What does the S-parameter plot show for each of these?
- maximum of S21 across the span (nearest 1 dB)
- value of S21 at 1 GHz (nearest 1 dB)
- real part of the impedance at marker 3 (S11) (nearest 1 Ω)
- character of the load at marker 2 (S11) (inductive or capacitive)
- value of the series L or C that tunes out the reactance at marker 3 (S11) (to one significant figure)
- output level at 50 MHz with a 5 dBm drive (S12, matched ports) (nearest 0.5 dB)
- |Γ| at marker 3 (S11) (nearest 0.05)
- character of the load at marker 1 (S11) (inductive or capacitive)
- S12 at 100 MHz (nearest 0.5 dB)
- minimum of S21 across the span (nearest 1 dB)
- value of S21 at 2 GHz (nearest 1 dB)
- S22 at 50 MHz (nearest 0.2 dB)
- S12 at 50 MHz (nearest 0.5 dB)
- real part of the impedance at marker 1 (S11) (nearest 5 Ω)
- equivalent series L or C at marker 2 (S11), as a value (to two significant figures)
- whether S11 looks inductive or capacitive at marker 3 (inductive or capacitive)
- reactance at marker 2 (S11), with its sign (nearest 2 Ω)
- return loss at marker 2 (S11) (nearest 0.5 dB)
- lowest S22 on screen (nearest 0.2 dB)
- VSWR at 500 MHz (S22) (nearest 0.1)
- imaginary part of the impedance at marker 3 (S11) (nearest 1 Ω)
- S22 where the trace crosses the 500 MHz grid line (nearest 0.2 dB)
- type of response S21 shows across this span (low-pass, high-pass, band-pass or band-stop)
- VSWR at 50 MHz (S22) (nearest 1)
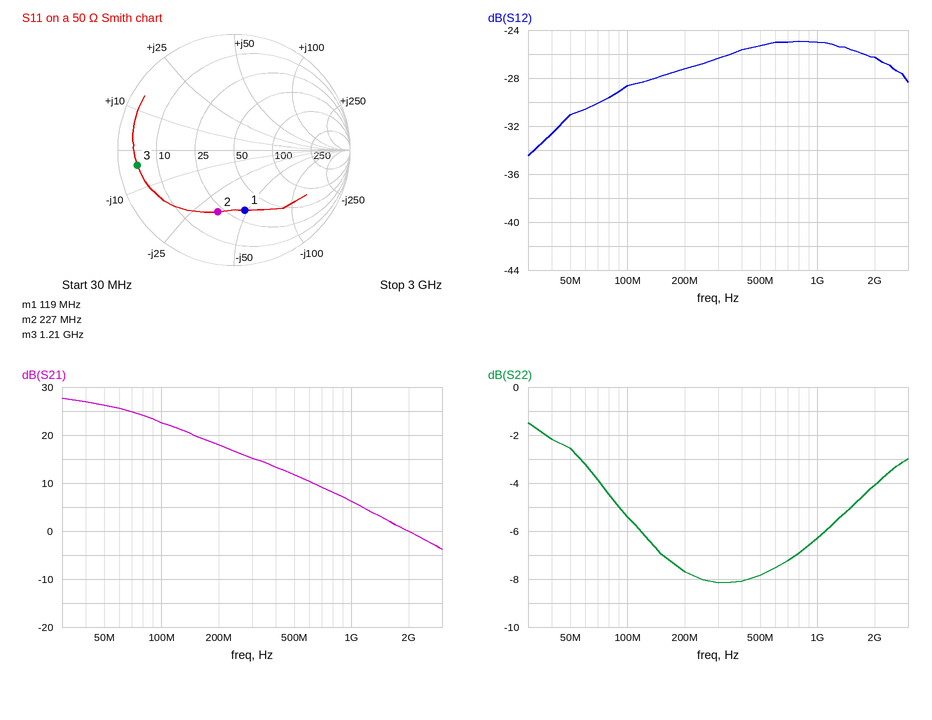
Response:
28 dB
6 dB
4 Ω
capacitive
500 pH
-26.0 dBm
0.85
capacitive
-28.5 dB
-4 dB
0 dB
-2.6 dB
-31.0 dB
35 Ω
21 pF
capacitive
-34 Ω
5.0 dB
-8.2 dB
2.4
-4 Ω
-7.8 dB
low-pass
7
